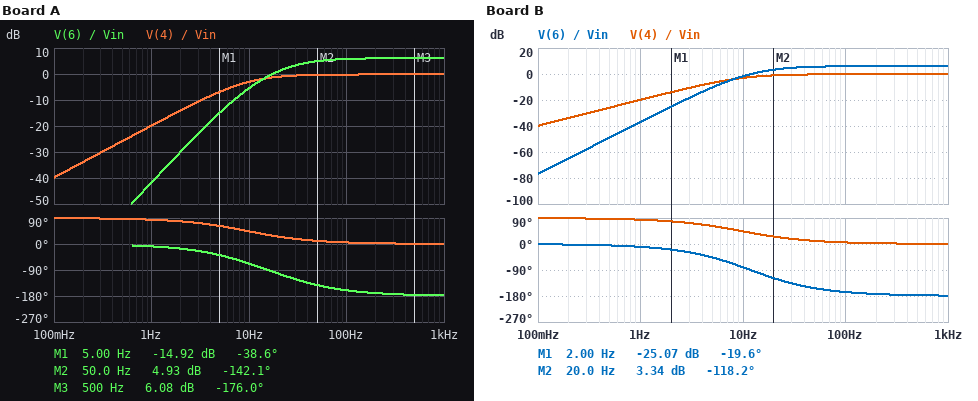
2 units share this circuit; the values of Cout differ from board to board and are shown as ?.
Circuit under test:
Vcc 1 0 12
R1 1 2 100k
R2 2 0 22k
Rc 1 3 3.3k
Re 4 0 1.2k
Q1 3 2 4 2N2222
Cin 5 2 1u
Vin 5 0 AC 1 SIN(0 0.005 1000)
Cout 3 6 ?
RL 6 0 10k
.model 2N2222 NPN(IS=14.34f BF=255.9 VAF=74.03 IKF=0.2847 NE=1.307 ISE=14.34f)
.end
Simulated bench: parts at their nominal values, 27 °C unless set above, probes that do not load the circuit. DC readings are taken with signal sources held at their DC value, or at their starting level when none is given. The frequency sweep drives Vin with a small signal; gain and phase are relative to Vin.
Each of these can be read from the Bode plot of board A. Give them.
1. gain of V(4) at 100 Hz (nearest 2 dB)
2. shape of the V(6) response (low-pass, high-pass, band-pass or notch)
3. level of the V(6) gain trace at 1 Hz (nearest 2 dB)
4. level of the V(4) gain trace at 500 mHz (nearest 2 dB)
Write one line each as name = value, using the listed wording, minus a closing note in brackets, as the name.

gain of V(4) at 100 Hz = 0 dB
shape of the V(6) response = high-pass
level of the V(6) gain trace at 1 Hz = -42 dB
level of the V(4) gain trace at 500 mHz = -26 dB
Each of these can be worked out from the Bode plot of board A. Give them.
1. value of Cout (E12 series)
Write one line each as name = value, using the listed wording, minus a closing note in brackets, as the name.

value of Cout = 470 nF
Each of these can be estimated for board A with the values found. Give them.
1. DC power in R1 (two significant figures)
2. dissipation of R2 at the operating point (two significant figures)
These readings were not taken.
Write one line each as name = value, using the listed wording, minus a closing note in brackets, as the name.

DC power in R1 = 990 µW
dissipation of R2 at the operating point = 190 µW
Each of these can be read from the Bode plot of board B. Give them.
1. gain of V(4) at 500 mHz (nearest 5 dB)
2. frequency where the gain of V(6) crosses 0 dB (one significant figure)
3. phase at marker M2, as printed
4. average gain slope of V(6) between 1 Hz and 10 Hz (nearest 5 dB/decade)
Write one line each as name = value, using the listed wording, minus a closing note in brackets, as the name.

gain of V(4) at 500 mHz = -25 dB
frequency where the gain of V(6) crosses 0 dB = 10 Hz
phase at marker M2, as printed = -118.2 deg
average gain slope of V(6) between 1 Hz and 10 Hz = 35 dB/decade
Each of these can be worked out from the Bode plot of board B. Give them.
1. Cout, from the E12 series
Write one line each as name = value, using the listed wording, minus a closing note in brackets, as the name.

Cout, from the E12 series = 820 nF
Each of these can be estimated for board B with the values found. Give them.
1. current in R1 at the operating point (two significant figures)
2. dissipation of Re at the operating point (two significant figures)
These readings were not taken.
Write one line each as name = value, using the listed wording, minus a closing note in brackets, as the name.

current in R1 at the operating point = 100 µA
dissipation of Re at the operating point = 1.6 mW
